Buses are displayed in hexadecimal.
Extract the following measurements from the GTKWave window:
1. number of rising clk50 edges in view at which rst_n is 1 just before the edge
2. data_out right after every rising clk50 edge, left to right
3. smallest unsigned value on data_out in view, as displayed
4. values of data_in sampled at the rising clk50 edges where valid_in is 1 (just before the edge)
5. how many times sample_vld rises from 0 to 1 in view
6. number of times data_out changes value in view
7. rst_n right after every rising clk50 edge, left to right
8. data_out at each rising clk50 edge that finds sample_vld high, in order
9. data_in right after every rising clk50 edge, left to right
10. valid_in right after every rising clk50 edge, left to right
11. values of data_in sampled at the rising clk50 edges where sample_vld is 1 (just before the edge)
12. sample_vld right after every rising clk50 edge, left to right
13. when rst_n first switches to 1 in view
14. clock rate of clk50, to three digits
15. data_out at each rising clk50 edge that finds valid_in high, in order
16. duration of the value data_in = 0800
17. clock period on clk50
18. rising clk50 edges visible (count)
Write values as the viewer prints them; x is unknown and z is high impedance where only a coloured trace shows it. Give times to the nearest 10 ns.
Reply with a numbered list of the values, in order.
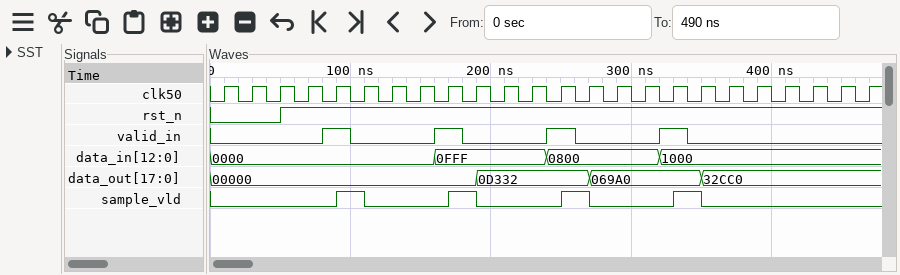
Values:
1. 21
2. 00000, 00000, 00000, 00000, 00000, 00000, 00000, 00000, 00000, 0D332, 0D332, 0D332, 0D332, 069A0, 069A0, 069A0, 069A0, 32CC0, 32CC0, 32CC0, 32CC0, 32CC0, 32CC0, 32CC0
3. 00000
4. 0000, 0FFF, 0800, 1000
5. 4
6. 3
7. 0 0 1 1 1 1 1 1 1 1 1 1 1 1 1 1 1 1 1 1 1 1 1 1
8. 00000, 00000, 0D332, 069A0
9. 0000, 0000, 0000, 0000, 0000, 0000, 0000, 0000, 0FFF, 0FFF, 0FFF, 0FFF, 0800, 0800, 0800, 0800, 1000, 1000, 1000, 1000, 1000, 1000, 1000, 1000
10. 0 0 0 0 1 0 0 0 1 0 0 0 1 0 0 0 1 0 0 0 0 0 0 0
11. 0000, 0FFF, 0800, 1000
12. 0 0 0 0 1 0 0 0 1 0 0 0 1 0 0 0 1 0 0 0 0 0 0 0
13. 50 ns
14. 50.0 MHz
15. 00000, 00000, 0D332, 069A0
16. 80 ns
17. 20 ns
18. 24
